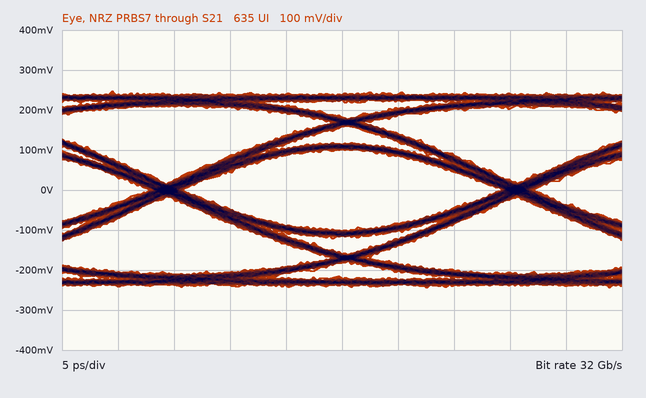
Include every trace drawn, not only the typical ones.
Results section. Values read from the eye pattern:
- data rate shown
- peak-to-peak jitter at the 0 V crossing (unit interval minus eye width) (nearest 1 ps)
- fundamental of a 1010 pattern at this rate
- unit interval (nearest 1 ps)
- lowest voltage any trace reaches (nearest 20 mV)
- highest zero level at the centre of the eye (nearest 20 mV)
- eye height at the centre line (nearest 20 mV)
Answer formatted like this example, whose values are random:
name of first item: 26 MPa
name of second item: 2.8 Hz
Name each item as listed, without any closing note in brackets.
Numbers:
data rate shown: 32 Gb/s
peak-to-peak jitter at the 0 V crossing (unit interval minus eye width): 3 ps
fundamental of a 1010 pattern at this rate: 16 GHz
unit interval: 31 ps
lowest voltage any trace reaches: -240 mV
highest zero level at the centre of the eye: -100 mV
eye height at the centre line: 200 mV
